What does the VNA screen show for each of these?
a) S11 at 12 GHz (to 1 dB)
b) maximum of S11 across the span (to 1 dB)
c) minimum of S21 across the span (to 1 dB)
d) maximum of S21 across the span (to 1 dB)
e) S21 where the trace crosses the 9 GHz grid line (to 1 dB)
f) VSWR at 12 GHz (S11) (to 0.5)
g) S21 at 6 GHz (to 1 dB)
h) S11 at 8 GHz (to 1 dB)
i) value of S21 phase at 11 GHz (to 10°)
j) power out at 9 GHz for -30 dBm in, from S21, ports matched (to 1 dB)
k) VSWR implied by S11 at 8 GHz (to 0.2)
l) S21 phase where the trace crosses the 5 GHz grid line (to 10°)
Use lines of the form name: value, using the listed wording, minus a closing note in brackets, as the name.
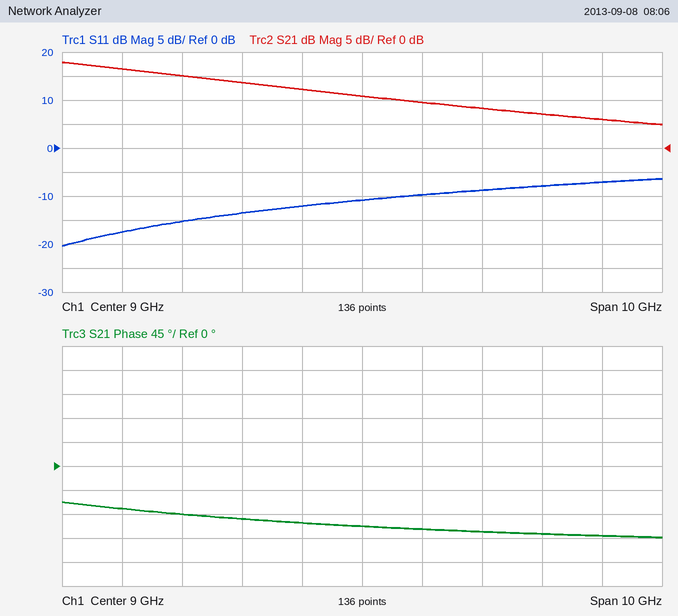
S11 at 12 GHz: -8 dB
maximum of S11 across the span: -6 dB
minimum of S21 across the span: 5 dB
maximum of S21 across the span: 18 dB
S21 where the trace crosses the 9 GHz grid line: 11 dB
VSWR at 12 GHz (S11): 2.5
S21 at 6 GHz: 15 dB
S11 at 8 GHz: -12 dB
value of S21 phase at 11 GHz: -120°
power out at 9 GHz for -30 dBm in, from S21, ports matched: -19 dBm
VSWR implied by S11 at 8 GHz: 1.6
S21 phase where the trace crosses the 5 GHz grid line: -80°
